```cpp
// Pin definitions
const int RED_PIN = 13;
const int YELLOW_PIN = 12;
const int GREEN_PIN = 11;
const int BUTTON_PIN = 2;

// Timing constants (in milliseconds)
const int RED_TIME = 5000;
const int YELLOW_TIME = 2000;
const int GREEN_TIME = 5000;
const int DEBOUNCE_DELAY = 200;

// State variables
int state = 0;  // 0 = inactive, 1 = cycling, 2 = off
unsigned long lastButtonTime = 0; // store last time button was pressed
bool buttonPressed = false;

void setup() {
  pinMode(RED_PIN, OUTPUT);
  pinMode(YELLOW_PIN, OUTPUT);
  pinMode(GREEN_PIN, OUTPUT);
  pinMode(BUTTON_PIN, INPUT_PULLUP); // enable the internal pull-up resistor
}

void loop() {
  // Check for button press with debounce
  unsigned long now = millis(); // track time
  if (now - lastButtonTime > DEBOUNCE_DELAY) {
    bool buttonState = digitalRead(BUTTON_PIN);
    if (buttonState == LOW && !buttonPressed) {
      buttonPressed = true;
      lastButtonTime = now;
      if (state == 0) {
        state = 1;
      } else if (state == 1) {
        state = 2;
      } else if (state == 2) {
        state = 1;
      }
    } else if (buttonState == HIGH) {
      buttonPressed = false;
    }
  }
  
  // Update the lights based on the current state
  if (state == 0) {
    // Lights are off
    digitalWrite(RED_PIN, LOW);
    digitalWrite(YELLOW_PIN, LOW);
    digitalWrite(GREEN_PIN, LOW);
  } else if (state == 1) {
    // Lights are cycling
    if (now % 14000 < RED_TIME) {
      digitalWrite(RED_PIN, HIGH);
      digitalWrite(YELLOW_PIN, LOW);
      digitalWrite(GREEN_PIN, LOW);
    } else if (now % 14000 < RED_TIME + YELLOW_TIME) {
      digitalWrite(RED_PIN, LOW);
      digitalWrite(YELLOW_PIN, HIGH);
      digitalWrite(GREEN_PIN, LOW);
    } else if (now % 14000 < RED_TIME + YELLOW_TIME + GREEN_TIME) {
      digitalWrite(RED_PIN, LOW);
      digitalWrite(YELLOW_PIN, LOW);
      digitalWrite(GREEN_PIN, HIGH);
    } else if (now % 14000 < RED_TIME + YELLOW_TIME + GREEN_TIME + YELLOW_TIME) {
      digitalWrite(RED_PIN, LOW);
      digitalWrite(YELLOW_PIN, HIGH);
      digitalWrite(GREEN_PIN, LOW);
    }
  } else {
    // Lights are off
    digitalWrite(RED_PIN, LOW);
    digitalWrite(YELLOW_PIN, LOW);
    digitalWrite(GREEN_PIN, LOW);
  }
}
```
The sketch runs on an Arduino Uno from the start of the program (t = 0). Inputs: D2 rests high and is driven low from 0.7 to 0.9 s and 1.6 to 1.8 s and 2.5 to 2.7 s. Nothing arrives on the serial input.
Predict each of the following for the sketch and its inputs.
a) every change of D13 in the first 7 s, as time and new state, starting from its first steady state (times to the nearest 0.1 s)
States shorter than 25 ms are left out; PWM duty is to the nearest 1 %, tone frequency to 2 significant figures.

0 s low; 0.7 s high; 1.6 s low; 2.5 s high; 5 s low
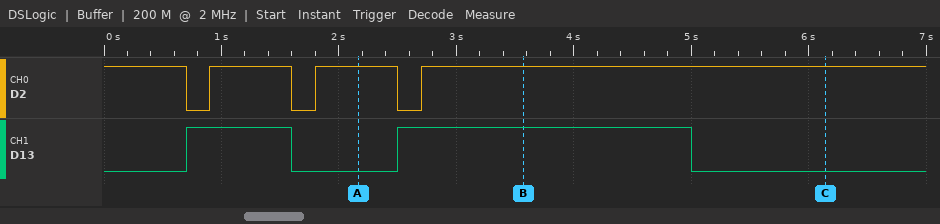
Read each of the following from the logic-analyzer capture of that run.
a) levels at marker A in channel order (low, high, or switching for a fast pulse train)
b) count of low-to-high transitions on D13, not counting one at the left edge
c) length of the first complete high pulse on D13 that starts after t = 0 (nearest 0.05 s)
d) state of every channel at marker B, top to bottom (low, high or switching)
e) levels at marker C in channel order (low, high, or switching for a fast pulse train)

D2 high, D13 low
2
0.90 s
D2 high, D13 high
D2 high, D13 low
